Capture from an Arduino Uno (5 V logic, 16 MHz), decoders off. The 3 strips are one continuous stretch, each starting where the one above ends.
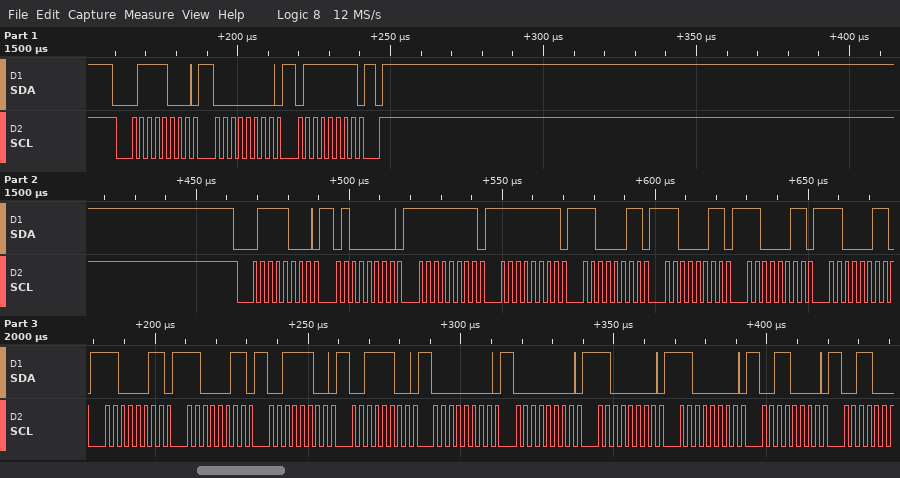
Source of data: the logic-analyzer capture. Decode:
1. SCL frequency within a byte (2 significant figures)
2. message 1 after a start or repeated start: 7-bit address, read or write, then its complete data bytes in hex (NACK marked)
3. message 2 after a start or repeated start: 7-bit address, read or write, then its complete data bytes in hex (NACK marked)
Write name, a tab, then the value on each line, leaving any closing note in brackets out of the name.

SCL frequency within a byte	400 kHz
message 1 after a start or repeated start: 7-bit address, read or write, then its complete data bytes in hex	0x3C write: 00 7F
message 2 after a start or repeated start: 7-bit address, read or write, then its complete data bytes in hex	0x3C write: 40 FF FF C3 C3 C3 C3 C3 C3 3C 3C 00 00 C0 C0 30
